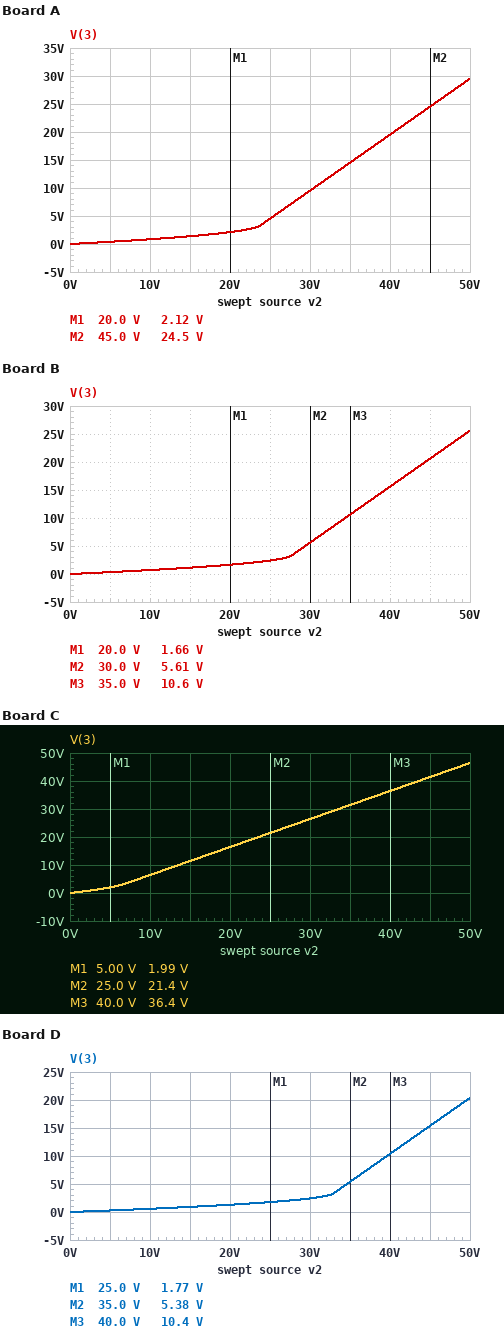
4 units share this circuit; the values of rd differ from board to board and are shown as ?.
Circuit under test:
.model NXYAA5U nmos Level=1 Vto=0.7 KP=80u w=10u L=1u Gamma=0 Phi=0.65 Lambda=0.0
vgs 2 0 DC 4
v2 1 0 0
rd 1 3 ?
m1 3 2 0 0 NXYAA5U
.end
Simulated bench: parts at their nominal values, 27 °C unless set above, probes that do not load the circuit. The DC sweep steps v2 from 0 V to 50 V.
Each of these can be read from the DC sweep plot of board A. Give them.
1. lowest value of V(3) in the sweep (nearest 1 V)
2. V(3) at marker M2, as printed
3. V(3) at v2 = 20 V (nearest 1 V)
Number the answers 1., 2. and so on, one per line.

1. 0 V
2. 24.5 V
3. 2 V
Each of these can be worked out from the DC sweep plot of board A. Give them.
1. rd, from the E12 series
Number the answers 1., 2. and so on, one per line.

1. 4.7 kΩ
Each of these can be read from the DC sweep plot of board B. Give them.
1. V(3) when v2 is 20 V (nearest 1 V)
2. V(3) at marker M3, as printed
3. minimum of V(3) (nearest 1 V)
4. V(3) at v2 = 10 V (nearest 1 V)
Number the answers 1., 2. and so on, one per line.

1. 2 V
2. 10.6 V
3. 0 V
4. 1 V
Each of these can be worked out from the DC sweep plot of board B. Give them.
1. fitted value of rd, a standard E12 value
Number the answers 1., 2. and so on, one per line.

1. 5.6 kΩ
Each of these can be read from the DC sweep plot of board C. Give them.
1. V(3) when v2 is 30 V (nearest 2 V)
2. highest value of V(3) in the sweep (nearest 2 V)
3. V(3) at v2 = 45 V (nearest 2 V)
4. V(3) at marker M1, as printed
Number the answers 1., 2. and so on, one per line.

1. 26 V
2. 46 V
3. 42 V
4. 1.99 V
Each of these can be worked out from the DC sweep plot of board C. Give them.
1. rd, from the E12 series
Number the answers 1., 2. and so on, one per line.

1. 820 Ω
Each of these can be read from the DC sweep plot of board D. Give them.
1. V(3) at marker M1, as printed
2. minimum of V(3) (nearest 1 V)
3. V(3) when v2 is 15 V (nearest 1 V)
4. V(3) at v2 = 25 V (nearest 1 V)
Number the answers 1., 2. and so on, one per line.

1. 1.77 V
2. 0 V
3. 1 V
4. 2 V
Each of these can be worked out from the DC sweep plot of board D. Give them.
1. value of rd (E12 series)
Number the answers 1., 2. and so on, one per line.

1. 6.8 kΩ
